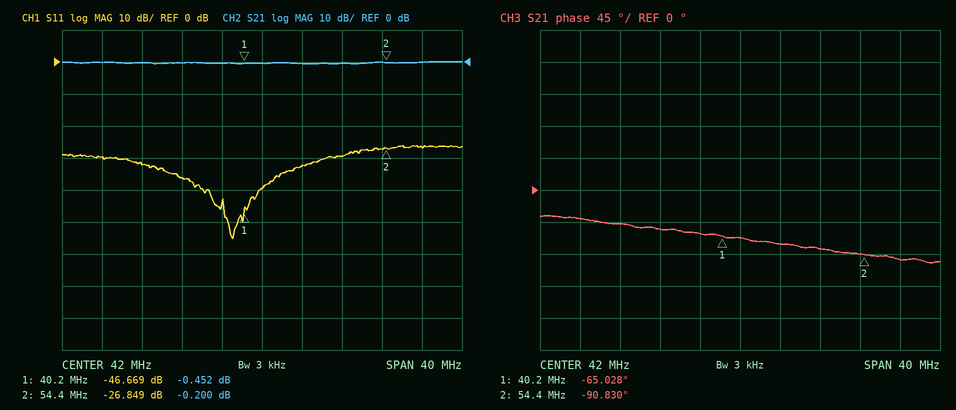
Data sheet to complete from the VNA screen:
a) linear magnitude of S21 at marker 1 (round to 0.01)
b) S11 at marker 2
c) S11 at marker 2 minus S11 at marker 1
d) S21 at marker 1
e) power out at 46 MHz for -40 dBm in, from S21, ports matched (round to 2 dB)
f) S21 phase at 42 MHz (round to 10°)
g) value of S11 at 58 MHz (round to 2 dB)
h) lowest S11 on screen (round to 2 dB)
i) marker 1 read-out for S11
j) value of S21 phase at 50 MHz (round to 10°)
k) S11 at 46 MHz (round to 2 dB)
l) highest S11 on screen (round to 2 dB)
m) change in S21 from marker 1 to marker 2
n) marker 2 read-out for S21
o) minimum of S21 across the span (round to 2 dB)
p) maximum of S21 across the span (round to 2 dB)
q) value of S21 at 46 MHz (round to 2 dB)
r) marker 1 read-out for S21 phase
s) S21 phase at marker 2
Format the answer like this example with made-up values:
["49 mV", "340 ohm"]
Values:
["0.95", "-26.849 dB", "19.820 dB", "-0.452 dB", "-40 dBm", "-70°", "-26 dB", "-56 dB", "-46.669 dB", "-80°", "-32 dB", "-26 dB", "0.252 dB", "-0.200 dB", "0 dB", "0 dB", "0 dB", "-65.028°", "-90.830°"]
